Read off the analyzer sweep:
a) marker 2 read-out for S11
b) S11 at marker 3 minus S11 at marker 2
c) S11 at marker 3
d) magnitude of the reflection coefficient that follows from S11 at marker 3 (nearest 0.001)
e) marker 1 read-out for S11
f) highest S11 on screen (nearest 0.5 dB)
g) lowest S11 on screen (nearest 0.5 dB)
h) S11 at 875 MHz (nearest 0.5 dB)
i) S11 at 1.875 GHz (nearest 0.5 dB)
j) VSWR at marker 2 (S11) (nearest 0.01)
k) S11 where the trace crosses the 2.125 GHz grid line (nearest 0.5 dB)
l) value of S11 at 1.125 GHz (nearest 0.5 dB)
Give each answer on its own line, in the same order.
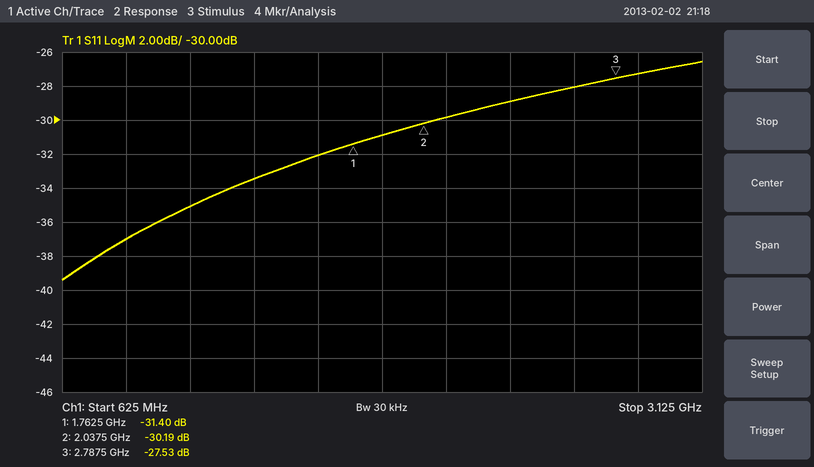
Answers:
-30.19 dB
2.66 dB
-27.53 dB
0.042
-31.40 dB
-26.5 dB
-39.5 dB
-37.0 dB
-31.0 dB
1.06
-30.0 dB
-35.0 dB
